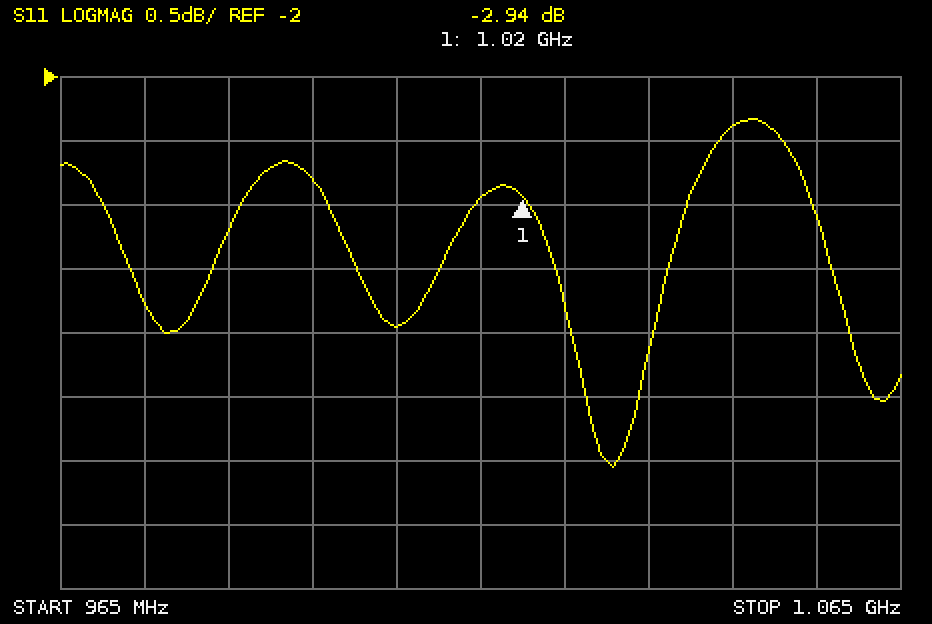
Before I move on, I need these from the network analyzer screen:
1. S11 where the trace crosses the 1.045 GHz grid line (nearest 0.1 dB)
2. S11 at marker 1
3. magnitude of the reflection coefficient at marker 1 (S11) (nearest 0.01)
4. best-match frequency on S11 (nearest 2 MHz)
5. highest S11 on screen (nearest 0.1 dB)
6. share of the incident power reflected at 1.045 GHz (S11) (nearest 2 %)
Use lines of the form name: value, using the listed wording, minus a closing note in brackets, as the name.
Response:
S11 where the trace crosses the 1.045 GHz grid line: -2.4 dB
S11 at marker 1: -2.94 dB
magnitude of the reflection coefficient at marker 1 (S11): 0.71
best-match frequency on S11: 1.030 GHz
highest S11 on screen: -2.3 dB
share of the incident power reflected at 1.045 GHz (S11): 58 %
